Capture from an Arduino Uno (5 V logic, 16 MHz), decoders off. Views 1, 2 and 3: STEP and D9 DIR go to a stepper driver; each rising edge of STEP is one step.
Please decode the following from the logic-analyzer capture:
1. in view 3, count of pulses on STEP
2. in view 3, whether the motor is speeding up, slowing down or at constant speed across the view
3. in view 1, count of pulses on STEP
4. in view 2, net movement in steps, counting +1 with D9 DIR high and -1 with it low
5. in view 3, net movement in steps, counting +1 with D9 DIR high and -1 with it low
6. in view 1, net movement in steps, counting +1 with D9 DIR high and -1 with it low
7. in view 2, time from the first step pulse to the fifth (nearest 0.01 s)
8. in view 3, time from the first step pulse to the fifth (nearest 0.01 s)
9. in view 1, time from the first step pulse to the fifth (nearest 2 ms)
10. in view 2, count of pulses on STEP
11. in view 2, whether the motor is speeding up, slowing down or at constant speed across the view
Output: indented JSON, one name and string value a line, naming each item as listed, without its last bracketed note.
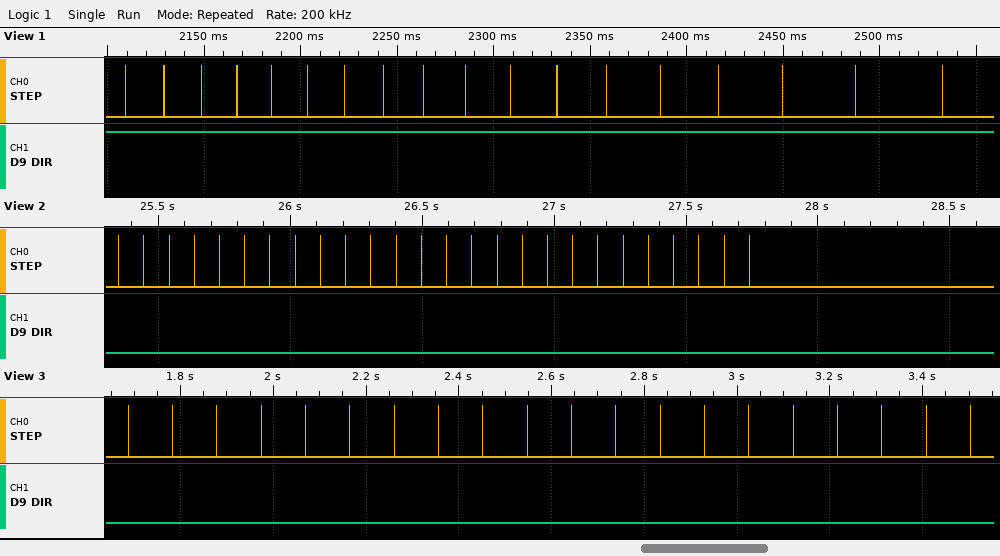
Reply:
{
  "in view 3, count of pulses on STEP": "20",
  "in view 3, whether the motor is speeding up, slowing down or at constant speed across the view": "constant speed",
  "in view 1, count of pulses on STEP": "18",
  "in view 2, net movement in steps, counting +1 with D9 DIR high and -1 with it low": "-26",
  "in view 3, net movement in steps, counting +1 with D9 DIR high and -1 with it low": "-20",
  "in view 1, net movement in steps, counting +1 with D9 DIR high and -1 with it low": "+18",
  "in view 2, time from the first step pulse to the fifth": "0.38 s",
  "in view 3, time from the first step pulse to the fifth": "0.38 s",
  "in view 1, time from the first step pulse to the fifth": "76 ms",
  "in view 2, count of pulses on STEP": "26",
  "in view 2, whether the motor is speeding up, slowing down or at constant speed across the view": "constant speed"
}
